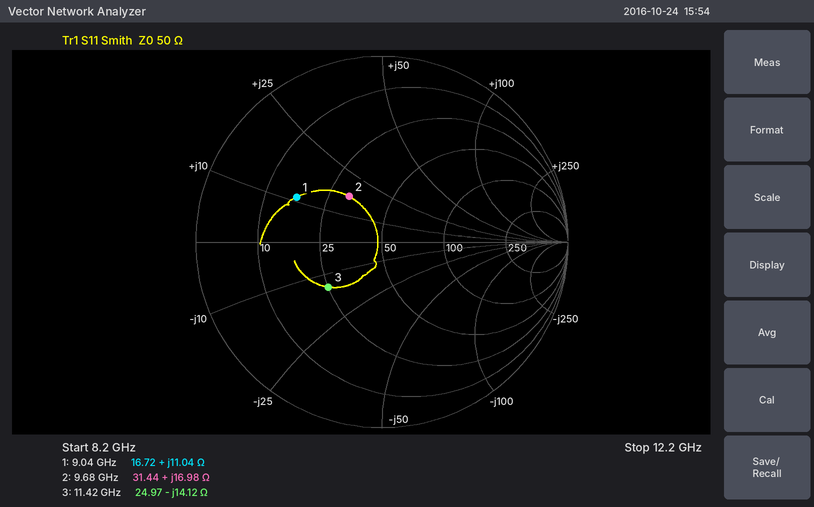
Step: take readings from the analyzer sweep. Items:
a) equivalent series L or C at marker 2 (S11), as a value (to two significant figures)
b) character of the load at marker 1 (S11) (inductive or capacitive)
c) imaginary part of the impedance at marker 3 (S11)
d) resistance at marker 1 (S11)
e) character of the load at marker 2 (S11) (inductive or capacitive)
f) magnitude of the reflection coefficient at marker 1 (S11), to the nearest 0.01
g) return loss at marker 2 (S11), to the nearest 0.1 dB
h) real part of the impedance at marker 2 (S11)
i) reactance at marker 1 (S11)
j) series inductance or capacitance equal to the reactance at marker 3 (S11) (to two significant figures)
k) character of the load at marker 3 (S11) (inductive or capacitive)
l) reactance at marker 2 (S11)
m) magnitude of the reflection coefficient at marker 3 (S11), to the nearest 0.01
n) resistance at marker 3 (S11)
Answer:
280 pH
inductive
-14.12 Ω
16.72 Ω
inductive
0.52
10.4 dB
31.44 Ω
+11.04 Ω
990 fF
capacitive
+16.98 Ω
0.38
24.97 Ω
